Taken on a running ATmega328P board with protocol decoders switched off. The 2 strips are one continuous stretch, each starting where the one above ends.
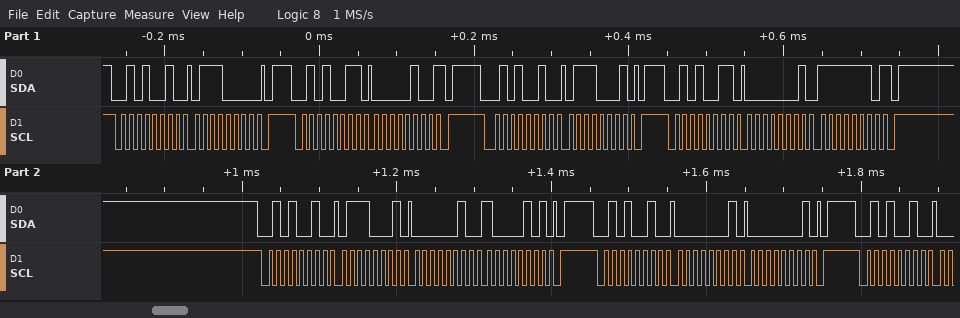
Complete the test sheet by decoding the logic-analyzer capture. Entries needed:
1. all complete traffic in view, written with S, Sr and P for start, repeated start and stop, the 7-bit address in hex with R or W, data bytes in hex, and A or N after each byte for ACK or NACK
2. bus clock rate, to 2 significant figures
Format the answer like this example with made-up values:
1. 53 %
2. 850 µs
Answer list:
1. S 29W A 70 A P S 29R A 04 N P S 29W A 71 A P S 29R A 01 A FE N P S 29W A 71 A 02 A 85 A P S 29W A 01 A 01 A P S 29W A
2. 100 kHz
